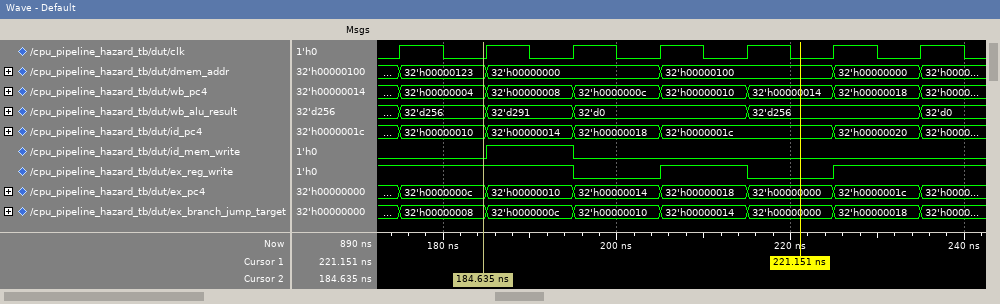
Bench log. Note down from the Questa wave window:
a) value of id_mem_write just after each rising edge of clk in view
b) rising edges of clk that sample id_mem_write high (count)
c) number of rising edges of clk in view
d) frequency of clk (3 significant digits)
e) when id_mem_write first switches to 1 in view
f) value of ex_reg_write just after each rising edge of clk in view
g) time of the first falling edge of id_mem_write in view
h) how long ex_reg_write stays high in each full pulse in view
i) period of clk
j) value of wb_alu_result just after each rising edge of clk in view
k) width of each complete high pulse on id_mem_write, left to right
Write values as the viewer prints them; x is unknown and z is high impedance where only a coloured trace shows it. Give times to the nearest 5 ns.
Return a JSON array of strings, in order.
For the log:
["0 1 0 0 0 0 0", "1", "7", "100 MHz", "185 ns", "1 1 0 1 0 1 1", "195 ns", "10 ns", "10 ns", "32'd256, 32'd291, 32'd0, 32'd0, 32'd256, 32'd256, 32'd0", "10 ns"]
